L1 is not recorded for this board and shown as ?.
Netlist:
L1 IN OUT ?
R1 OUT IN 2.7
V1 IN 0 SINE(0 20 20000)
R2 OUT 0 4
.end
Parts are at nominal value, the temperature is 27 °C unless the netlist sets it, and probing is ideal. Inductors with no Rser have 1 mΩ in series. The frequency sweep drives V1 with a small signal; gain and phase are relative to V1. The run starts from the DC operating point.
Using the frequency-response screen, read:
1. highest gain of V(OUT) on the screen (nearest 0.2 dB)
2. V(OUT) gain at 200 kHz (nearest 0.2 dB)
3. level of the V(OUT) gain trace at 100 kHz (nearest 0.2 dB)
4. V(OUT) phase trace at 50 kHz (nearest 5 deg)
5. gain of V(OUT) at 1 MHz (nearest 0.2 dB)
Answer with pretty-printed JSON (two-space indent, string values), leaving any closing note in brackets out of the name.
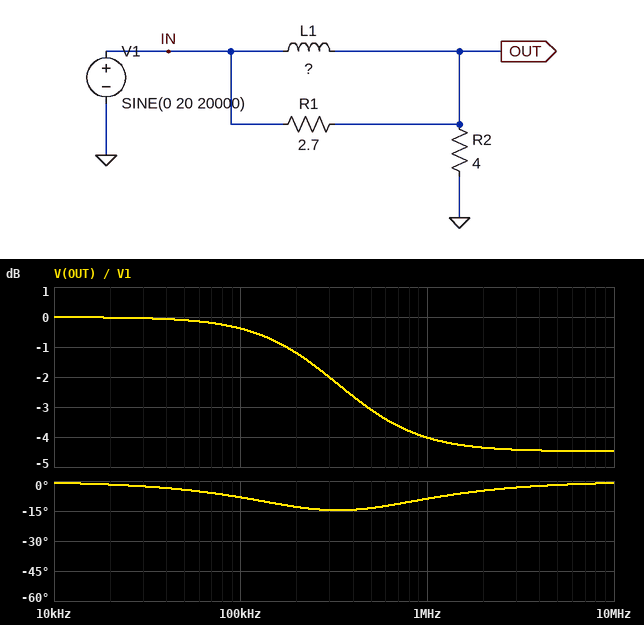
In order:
{
  "highest gain of V(OUT) on the screen": "0 dB",
  "V(OUT) gain at 200 kHz": "-1.2 dB",
  "level of the V(OUT) gain trace at 100 kHz": "-0.4 dB",
  "V(OUT) phase trace at 50 kHz": "-5 deg",
  "gain of V(OUT) at 1 MHz": "-4.0 dB"
}
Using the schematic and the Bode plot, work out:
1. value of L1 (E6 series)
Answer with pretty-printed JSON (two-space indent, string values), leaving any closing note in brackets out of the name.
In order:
{
  "value of L1": "1 µH"
}
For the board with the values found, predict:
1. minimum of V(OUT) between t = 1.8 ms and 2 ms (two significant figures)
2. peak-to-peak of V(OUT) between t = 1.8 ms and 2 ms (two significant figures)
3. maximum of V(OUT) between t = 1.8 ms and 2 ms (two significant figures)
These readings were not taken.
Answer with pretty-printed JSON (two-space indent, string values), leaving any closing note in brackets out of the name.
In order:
{
  "minimum of V(OUT) between t = 1.8 ms and 2 ms": "-20 V",
  "peak-to-peak of V(OUT) between t = 1.8 ms and 2 ms": "40 V",
  "maximum of V(OUT) between t = 1.8 ms and 2 ms": "20 V"
}
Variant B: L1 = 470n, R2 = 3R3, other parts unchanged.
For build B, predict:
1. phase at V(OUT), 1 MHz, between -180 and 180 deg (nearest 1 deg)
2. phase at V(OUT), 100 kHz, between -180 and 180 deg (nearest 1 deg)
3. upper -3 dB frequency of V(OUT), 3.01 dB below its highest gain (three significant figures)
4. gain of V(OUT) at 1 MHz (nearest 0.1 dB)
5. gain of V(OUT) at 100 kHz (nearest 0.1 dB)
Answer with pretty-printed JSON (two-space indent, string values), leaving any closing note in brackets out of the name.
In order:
{
  "phase at V(OUT), 1 MHz, between -180 and 180 deg": "-16 deg",
  "phase at V(OUT), 100 kHz, between -180 and 180 deg": "-5 deg",
  "upper -3 dB frequency of V(OUT), 3.01 dB below its highest gain": "801 kHz",
  "gain of V(OUT) at 1 MHz": "-3.5 dB",
  "gain of V(OUT) at 100 kHz": "-0.1 dB"
}
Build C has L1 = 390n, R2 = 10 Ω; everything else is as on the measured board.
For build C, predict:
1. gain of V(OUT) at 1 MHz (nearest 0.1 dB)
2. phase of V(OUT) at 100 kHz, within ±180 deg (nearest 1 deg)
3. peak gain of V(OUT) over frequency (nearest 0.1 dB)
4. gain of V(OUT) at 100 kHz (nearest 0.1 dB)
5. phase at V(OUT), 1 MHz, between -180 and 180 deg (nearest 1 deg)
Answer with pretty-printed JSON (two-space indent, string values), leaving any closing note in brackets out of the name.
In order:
{
  "gain of V(OUT) at 1 MHz": "-1.1 dB",
  "phase of V(OUT) at 100 kHz, within ±180 deg": "-1 deg",
  "peak gain of V(OUT) over frequency": "0 dB",
  "gain of V(OUT) at 100 kHz": "0 dB",
  "phase at V(OUT), 1 MHz, between -180 and 180 deg": "-7 deg"
}
